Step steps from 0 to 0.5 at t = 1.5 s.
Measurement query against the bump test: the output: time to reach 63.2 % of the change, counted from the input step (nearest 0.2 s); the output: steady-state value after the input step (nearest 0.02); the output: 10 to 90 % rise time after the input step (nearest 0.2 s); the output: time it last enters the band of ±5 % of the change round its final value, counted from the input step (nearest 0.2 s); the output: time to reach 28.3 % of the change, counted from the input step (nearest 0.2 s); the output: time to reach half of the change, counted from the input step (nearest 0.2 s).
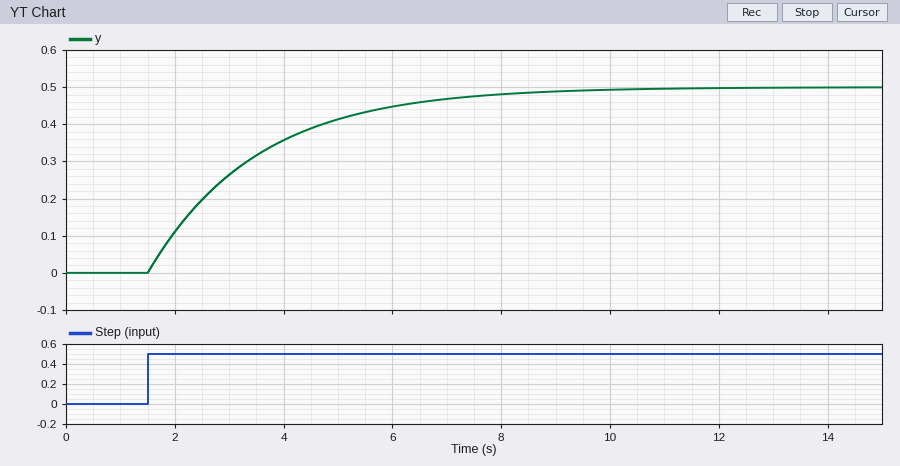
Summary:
2.0 s
0.50
4.4 s
6.0 s
0.6 s
1.4 s
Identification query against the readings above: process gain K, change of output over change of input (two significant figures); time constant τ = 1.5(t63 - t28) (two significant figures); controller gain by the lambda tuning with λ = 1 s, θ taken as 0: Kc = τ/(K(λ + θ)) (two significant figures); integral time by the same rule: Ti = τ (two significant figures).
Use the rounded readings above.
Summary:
1.0
2.1 s
2.1
2.1 s
